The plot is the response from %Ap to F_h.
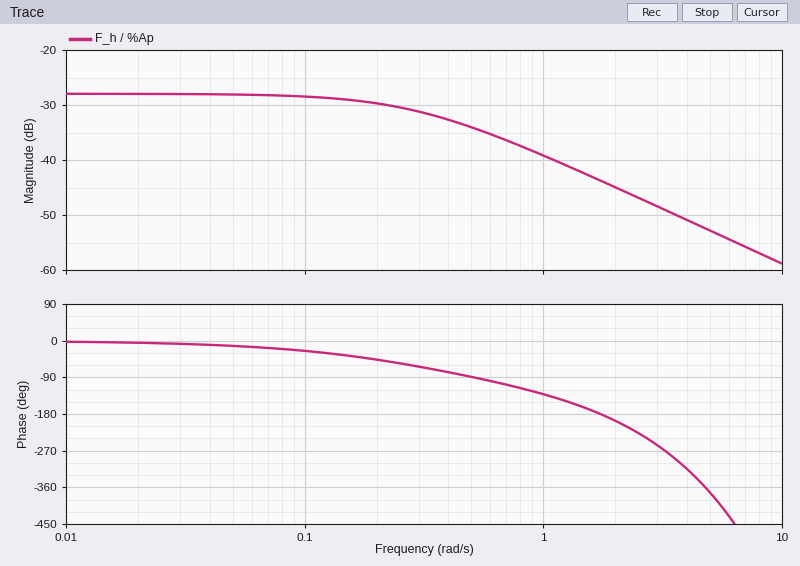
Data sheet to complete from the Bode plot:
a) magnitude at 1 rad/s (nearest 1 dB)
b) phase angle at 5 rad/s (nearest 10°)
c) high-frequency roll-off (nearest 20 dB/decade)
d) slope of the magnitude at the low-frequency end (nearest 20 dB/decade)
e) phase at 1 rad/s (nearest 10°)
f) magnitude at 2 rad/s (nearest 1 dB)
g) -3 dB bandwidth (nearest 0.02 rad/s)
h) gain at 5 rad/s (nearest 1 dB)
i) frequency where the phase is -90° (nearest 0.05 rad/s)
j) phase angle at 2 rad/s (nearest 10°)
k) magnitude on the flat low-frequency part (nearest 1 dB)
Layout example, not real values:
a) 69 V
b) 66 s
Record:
a) -39 dB
b) -370°
c) -20 dB/decade
d) 0 dB/decade
e) -130°
f) -45 dB
g) 0.28 rad/s
h) -53 dB
i) 0.50 rad/s
j) -200°
k) -28 dB
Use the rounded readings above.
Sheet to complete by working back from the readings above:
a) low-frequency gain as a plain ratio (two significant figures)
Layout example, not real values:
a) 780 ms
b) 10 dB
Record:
a) 0.040
